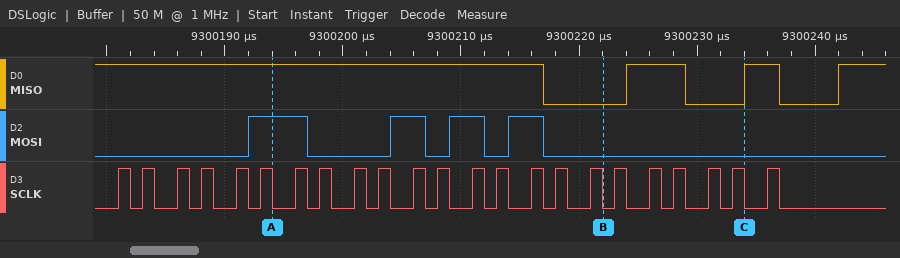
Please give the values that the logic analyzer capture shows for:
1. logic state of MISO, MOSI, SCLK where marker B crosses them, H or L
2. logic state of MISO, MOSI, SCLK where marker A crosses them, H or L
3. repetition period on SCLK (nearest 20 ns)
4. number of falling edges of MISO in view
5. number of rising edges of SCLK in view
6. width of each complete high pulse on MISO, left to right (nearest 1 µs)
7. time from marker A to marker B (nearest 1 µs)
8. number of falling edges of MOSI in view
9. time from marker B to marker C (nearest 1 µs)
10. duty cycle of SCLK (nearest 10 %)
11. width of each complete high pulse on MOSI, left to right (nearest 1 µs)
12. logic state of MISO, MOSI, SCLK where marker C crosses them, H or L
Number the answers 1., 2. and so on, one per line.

1. MISO=L, MOSI=L, SCLK=L
2. MISO=H, MOSI=H, SCLK=L
3. 2500 ns
4. 3
5. 23
6. 5 µs, 3 µs
7. 28 µs
8. 4
9. 12 µs
10. 40 %
11. 5 µs, 3 µs, 3 µs, 3 µs
12. MISO=H, MOSI=L, SCLK=L
